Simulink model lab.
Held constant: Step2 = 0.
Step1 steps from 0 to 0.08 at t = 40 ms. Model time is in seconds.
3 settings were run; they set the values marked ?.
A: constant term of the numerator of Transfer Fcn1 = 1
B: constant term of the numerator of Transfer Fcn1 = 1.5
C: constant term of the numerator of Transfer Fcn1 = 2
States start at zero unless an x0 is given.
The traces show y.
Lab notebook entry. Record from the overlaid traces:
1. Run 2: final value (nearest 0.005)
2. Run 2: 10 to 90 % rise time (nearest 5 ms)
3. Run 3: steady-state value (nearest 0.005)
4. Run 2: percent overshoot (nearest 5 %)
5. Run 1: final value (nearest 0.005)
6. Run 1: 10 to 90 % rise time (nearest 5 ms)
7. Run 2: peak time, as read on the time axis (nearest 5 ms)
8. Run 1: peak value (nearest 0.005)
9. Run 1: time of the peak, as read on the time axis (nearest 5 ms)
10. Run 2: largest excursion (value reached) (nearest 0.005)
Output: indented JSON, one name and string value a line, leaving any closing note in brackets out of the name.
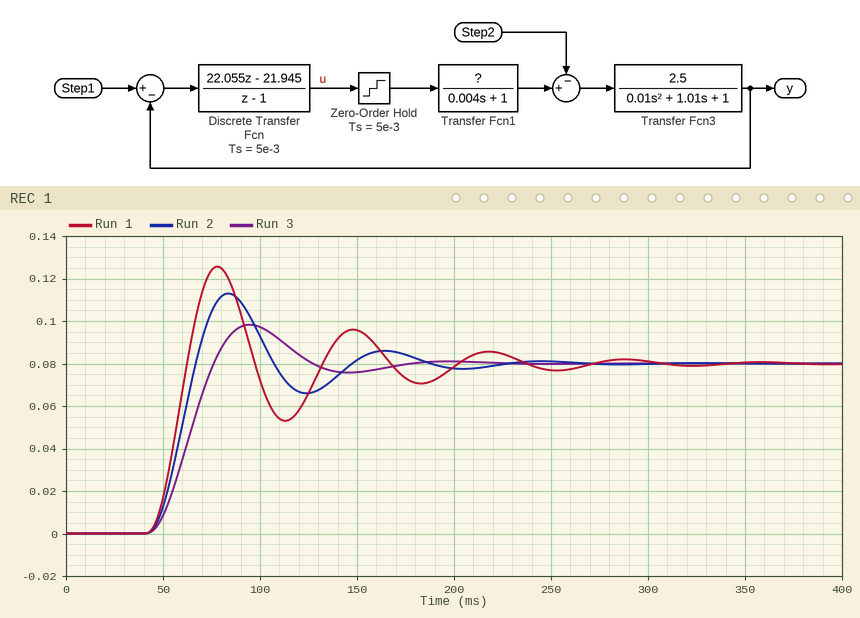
{
  "Run 2: final value": "0.080",
  "Run 2: 10 to 90 % rise time": "15 ms",
  "Run 3: steady-state value": "0.080",
  "Run 2: percent overshoot": "40 %",
  "Run 1: final value": "0.080",
  "Run 1: 10 to 90 % rise time": "15 ms",
  "Run 2: peak time, as read on the time axis": "85 ms",
  "Run 1: peak value": "0.125",
  "Run 1: time of the peak, as read on the time axis": "80 ms",
  "Run 2: largest excursion (value reached)": "0.115"
}
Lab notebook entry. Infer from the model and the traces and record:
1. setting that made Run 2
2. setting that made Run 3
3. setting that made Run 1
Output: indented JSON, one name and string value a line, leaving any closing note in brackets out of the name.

{
  "setting that made Run 2": "B",
  "setting that made Run 3": "A",
  "setting that made Run 1": "C"
}
